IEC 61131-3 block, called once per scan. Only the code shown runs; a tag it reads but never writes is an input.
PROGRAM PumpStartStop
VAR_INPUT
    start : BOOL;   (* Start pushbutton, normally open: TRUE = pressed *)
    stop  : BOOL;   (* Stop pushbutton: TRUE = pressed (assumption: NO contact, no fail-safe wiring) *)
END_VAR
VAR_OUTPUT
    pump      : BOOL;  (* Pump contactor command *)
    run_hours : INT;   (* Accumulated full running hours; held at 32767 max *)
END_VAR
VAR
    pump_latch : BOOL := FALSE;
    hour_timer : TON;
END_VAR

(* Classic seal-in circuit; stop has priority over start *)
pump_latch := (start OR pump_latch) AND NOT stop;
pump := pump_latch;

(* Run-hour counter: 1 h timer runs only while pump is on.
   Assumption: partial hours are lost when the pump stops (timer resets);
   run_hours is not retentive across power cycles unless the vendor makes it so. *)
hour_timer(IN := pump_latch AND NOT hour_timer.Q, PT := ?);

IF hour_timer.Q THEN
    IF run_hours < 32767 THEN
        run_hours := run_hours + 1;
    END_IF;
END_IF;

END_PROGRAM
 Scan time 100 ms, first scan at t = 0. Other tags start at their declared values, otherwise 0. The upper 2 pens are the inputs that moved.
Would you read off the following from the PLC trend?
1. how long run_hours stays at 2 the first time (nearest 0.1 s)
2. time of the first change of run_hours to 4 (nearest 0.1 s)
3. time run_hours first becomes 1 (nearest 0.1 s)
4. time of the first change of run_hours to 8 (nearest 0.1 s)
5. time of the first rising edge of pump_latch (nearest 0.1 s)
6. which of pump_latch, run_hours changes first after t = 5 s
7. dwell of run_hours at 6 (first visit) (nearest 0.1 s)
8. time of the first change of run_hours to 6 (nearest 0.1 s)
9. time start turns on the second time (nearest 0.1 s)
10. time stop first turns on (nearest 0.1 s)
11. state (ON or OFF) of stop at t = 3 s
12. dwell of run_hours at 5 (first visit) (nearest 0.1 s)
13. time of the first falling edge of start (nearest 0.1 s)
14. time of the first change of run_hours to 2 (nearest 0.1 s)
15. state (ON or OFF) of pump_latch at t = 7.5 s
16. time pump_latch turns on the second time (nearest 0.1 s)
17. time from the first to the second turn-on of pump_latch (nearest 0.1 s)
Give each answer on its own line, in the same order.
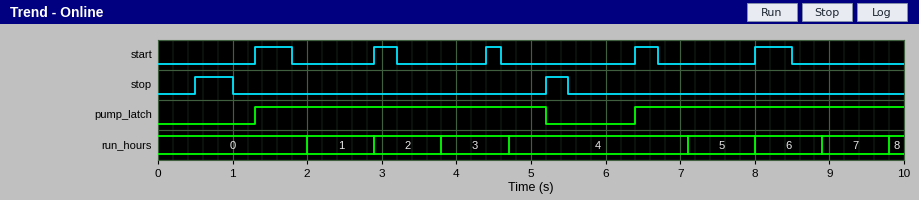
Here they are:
0.9 s
4.7 s
2.0 s
9.8 s
1.3 s
pump_latch
0.9 s
8.0 s
2.9 s
0.5 s
OFF
0.9 s
1.8 s
2.9 s
ON
6.4 s
5.1 s
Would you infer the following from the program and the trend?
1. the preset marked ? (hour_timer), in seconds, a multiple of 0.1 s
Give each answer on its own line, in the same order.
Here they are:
0.7 s
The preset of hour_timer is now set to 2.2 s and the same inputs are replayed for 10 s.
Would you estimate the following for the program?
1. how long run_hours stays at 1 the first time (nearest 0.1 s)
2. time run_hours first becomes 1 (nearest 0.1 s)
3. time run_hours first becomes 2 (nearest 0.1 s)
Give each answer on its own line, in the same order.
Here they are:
5.1 s
3.5 s
8.6 s
